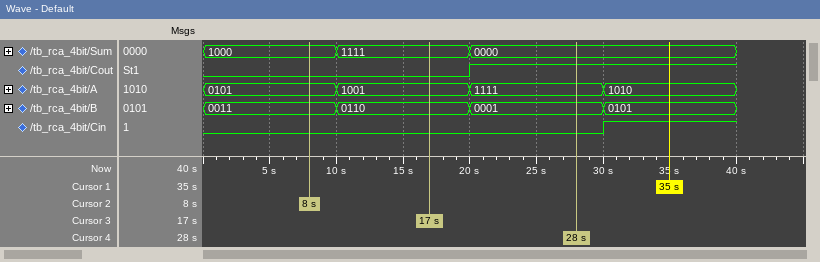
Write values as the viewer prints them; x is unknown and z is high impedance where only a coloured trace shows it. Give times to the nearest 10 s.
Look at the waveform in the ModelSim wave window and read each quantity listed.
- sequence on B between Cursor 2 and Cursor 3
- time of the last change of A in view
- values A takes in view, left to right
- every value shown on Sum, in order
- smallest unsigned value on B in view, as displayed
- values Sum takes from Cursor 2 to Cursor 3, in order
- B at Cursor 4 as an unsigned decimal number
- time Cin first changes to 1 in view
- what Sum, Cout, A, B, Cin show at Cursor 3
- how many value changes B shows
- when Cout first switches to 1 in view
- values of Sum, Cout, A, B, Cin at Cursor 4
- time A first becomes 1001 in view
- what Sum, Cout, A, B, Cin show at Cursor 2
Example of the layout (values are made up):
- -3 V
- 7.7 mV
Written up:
- 0011, 0110
- 30 s
- 0101, 1001, 1111, 1010
- 1000, 1111, 0000
- 0001
- 1000, 1111
- 1
- 30 s
- Sum=1111, Cout=0, A=1001, B=0110, Cin=0
- 3
- 20 s
- Sum=0000, Cout=1, A=1111, B=0001, Cin=0
- 10 s
- Sum=1000, Cout=0, A=0101, B=0011, Cin=0
